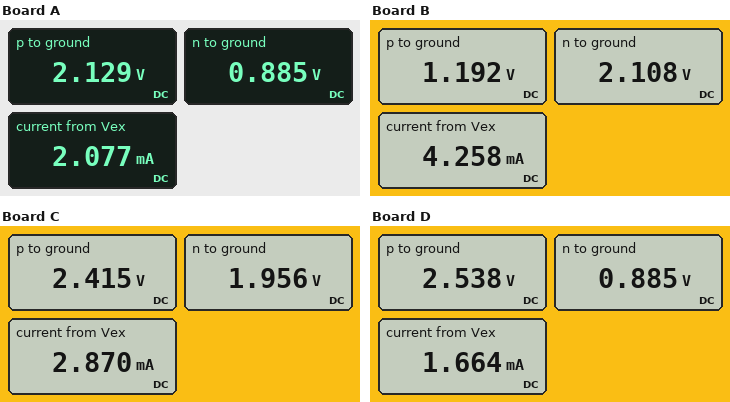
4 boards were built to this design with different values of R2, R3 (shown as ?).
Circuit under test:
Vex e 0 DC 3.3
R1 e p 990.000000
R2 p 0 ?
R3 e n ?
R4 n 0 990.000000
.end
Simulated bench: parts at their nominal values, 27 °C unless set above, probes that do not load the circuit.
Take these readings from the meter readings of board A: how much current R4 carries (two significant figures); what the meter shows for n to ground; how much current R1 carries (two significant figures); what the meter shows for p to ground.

890 µA
0.885 V
1.2 mA
2.129 V
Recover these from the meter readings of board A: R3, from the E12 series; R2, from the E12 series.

2.7 kΩ
1.8 kΩ
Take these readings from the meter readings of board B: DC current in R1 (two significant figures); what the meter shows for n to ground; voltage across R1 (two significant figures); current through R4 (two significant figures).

2.1 mA
2.108 V
2.1 V
2.1 mA
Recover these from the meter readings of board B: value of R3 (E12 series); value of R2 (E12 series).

560 Ω
560 Ω
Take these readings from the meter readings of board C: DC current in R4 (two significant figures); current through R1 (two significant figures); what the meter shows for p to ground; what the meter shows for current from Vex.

2.0 mA
890 µA
2.415 V
2.870 mA
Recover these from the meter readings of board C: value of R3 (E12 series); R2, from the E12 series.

680 Ω
2.7 kΩ
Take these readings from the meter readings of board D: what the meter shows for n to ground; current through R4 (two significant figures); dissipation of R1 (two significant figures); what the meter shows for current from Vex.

0.885 V
890 µA
590 µW
1.664 mA
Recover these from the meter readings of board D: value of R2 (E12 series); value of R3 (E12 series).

3.3 kΩ
2.7 kΩ
